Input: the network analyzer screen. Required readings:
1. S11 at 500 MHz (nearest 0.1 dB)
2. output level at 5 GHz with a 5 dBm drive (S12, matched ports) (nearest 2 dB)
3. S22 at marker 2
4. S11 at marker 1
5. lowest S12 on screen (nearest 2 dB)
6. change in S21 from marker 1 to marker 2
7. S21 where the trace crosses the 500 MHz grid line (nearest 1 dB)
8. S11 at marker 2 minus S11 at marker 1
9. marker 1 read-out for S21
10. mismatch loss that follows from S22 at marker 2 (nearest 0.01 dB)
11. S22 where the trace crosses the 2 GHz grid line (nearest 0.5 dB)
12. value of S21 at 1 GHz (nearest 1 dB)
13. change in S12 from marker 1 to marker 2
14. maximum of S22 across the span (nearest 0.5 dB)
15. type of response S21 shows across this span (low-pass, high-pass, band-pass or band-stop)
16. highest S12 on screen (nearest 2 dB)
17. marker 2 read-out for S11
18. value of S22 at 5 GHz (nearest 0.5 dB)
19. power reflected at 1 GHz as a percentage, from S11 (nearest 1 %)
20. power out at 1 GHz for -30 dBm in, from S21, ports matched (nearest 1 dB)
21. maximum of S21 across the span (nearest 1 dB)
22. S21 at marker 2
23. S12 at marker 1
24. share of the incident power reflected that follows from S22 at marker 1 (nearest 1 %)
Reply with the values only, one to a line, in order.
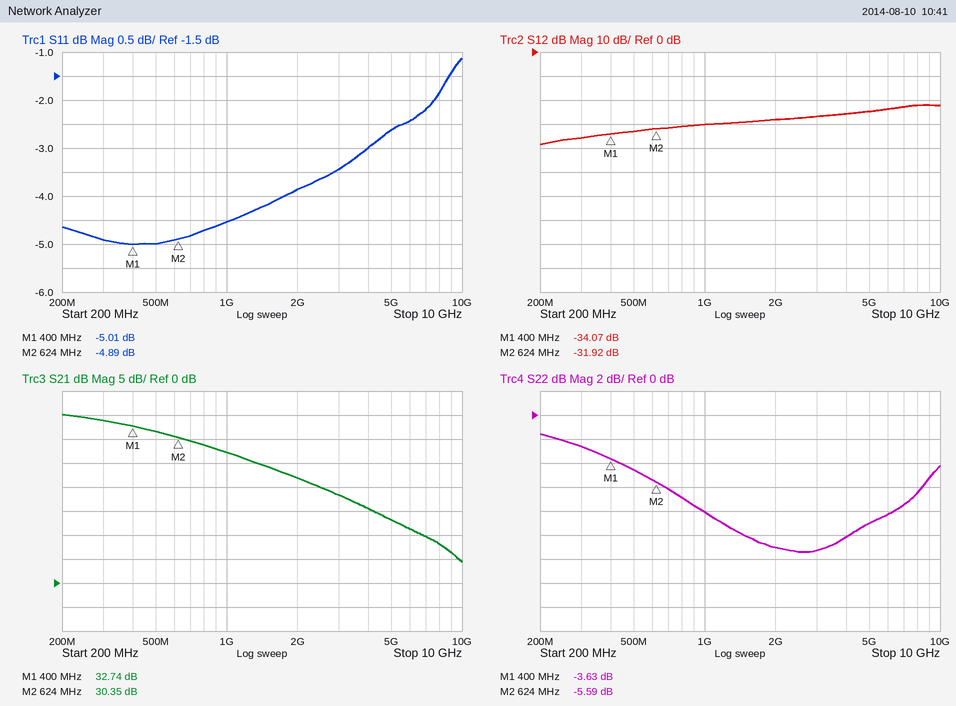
-5.0 dB
-20 dBm
-5.59 dB
-5.01 dB
-38 dB
-2.39 dB
32 dB
0.12 dB
32.74 dB
1.40 dB
-11.0 dB
27 dB
2.15 dB
-1.5 dB
low-pass
-22 dB
-4.89 dB
-9.0 dB
35 %
-3 dBm
35 dB
30.35 dB
-34.07 dB
43 %
